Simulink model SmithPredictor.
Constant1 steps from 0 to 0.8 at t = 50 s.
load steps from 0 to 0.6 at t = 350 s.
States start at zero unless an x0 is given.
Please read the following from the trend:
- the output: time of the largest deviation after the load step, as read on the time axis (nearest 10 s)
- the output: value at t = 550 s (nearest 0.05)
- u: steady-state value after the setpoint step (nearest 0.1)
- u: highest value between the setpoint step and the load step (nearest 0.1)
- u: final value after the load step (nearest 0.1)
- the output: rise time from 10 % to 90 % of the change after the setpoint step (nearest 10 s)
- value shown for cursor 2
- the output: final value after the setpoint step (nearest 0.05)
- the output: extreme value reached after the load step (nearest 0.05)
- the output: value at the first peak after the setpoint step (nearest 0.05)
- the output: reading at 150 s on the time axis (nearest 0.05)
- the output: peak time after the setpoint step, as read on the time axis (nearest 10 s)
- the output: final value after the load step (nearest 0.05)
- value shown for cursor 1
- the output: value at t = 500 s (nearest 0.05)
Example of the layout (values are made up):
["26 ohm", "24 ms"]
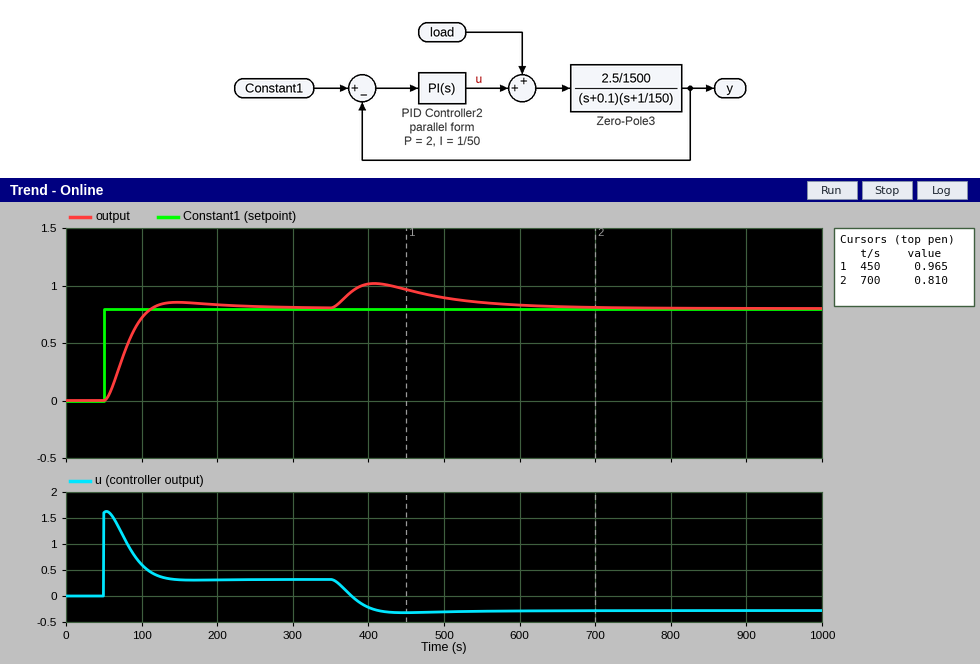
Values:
["410 s", "0.85", "0.3", "1.6", "-0.3", "40 s", "0.810", "0.80", "1.00", "0.85", "0.85", "150 s", "0.80", "0.965", "0.90"]
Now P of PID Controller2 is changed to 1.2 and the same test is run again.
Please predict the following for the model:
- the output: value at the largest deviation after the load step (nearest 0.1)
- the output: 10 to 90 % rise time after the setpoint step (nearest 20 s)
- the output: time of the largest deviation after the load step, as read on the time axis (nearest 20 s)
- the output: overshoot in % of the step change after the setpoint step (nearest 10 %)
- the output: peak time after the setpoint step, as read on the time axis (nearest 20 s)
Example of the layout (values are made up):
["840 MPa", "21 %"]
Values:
["1.1", "60 s", "420 s", "20 %", "180 s"]
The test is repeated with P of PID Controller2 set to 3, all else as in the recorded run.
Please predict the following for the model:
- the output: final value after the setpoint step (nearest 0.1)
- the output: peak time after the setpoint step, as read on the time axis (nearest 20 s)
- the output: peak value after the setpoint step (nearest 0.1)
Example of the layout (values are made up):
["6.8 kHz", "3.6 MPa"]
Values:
["0.8", "120 s", "0.8"]
